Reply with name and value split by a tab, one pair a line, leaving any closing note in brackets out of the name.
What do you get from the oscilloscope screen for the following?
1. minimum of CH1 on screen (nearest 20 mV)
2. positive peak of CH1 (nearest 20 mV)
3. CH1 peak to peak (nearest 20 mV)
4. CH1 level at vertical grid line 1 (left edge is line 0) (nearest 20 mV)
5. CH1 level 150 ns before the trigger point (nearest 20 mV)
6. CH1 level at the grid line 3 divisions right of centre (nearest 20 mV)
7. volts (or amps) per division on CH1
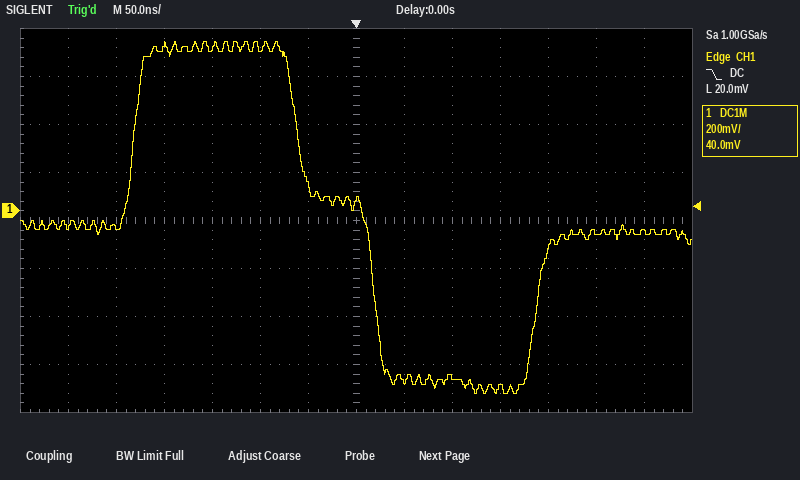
minimum of CH1 on screen	-760 mV
positive peak of CH1	700 mV
CH1 peak to peak	1.46 V
CH1 level at vertical grid line 1 (left edge is line 0)	-60 mV
CH1 level 150 ns before the trigger point	680 mV
CH1 level at the grid line 3 divisions right of centre	-740 mV
volts (or amps) per division on CH1	200 mV
